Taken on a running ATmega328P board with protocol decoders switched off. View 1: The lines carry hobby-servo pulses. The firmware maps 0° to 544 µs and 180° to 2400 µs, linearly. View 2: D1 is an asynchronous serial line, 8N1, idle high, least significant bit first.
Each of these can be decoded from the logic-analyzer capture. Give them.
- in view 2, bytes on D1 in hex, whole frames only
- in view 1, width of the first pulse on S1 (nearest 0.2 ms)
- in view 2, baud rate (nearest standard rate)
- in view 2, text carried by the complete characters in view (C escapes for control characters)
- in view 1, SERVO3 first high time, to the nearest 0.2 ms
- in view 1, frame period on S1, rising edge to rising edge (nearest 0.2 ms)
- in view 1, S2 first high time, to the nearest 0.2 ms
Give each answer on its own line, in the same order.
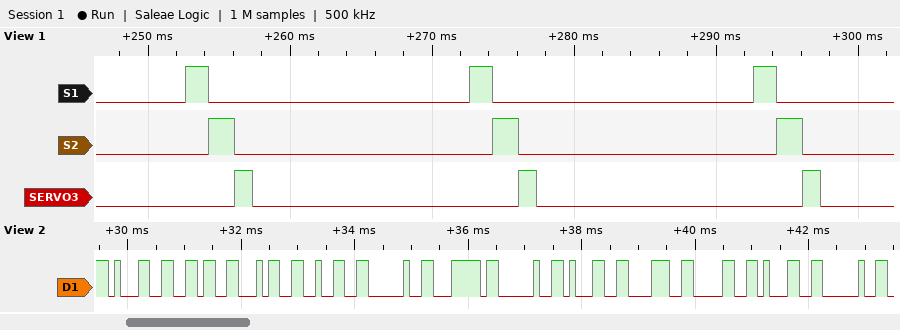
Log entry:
31 36 34 32 20 7C 20 31 38 30 31 20
1.6 ms
9600 baud
"1642 | 1801 "
1.2 ms
20.0 ms
1.8 ms
